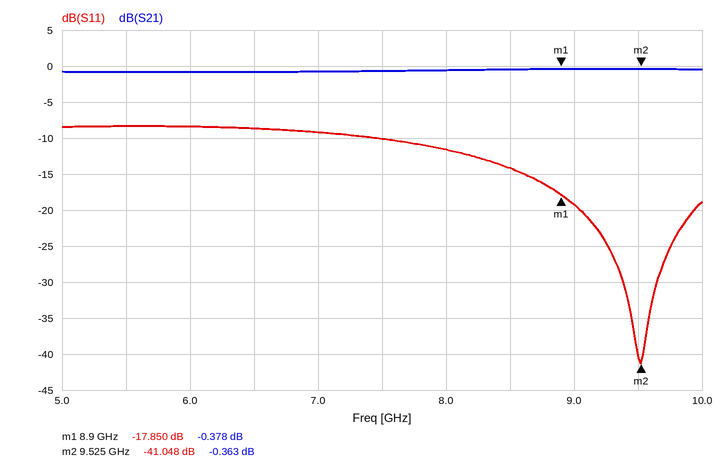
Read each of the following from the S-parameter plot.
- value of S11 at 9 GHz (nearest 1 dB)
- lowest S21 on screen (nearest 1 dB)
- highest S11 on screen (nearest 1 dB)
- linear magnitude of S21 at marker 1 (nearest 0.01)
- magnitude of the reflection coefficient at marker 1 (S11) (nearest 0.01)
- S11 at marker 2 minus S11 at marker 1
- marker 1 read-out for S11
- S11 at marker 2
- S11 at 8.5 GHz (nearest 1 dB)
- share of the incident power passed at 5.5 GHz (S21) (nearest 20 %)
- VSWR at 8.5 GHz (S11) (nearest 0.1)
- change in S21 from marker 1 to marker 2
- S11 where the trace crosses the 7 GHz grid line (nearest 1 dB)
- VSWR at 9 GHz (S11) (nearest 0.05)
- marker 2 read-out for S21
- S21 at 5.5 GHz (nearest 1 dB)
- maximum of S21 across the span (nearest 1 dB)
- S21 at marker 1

-19 dB
-1 dB
-8 dB
0.96
0.13
-23.198 dB
-17.850 dB
-41.048 dB
-14 dB
80 %
1.5
0.015 dB
-9 dB
1.25
-0.363 dB
-1 dB
0 dB
-0.378 dB
